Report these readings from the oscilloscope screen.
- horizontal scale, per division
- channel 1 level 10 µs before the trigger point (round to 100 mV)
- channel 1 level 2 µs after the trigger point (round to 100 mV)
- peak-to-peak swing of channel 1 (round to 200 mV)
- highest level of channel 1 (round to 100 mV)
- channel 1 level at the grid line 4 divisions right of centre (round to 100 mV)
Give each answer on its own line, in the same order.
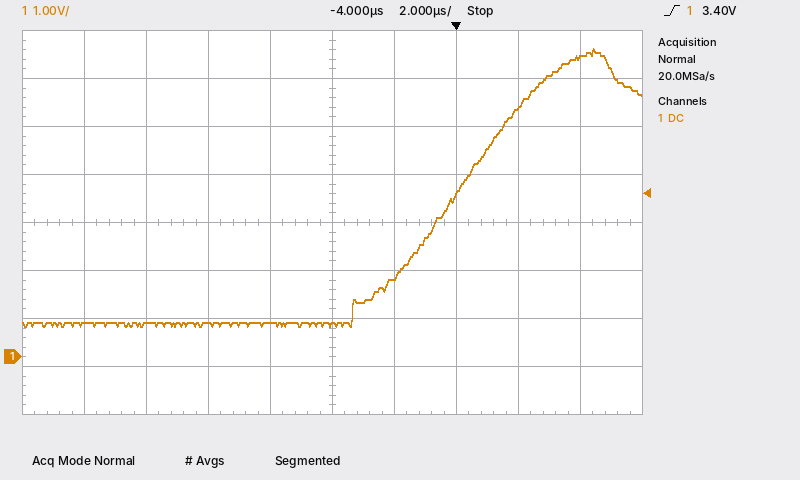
2 µs
700 mV
5.2 V
5.8 V
6.4 V
6.2 V
